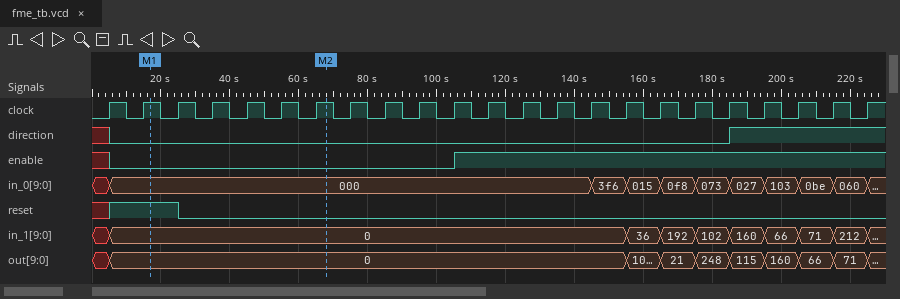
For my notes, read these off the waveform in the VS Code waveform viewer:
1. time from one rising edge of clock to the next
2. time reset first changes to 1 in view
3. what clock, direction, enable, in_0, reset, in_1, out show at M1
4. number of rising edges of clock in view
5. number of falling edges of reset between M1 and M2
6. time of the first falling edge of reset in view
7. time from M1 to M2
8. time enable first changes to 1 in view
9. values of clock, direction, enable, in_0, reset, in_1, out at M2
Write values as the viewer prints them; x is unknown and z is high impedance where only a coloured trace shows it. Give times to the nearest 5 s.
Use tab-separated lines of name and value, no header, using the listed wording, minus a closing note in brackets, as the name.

time from one rising edge of clock to the next	10 s
time reset first changes to 1 in view	5 s
what clock, direction, enable, in_0, reset, in_1, out show at M1	clock=1, direction=0, enable=0, in_0=000, reset=1, in_1=0, out=0
number of rising edges of clock in view	23
number of falling edges of reset between M1 and M2	1
time of the first falling edge of reset in view	25 s
time from M1 to M2	50 s
time enable first changes to 1 in view	105 s
values of clock, direction, enable, in_0, reset, in_1, out at M2	clock=1, direction=0, enable=0, in_0=000, reset=0, in_1=0, out=0
